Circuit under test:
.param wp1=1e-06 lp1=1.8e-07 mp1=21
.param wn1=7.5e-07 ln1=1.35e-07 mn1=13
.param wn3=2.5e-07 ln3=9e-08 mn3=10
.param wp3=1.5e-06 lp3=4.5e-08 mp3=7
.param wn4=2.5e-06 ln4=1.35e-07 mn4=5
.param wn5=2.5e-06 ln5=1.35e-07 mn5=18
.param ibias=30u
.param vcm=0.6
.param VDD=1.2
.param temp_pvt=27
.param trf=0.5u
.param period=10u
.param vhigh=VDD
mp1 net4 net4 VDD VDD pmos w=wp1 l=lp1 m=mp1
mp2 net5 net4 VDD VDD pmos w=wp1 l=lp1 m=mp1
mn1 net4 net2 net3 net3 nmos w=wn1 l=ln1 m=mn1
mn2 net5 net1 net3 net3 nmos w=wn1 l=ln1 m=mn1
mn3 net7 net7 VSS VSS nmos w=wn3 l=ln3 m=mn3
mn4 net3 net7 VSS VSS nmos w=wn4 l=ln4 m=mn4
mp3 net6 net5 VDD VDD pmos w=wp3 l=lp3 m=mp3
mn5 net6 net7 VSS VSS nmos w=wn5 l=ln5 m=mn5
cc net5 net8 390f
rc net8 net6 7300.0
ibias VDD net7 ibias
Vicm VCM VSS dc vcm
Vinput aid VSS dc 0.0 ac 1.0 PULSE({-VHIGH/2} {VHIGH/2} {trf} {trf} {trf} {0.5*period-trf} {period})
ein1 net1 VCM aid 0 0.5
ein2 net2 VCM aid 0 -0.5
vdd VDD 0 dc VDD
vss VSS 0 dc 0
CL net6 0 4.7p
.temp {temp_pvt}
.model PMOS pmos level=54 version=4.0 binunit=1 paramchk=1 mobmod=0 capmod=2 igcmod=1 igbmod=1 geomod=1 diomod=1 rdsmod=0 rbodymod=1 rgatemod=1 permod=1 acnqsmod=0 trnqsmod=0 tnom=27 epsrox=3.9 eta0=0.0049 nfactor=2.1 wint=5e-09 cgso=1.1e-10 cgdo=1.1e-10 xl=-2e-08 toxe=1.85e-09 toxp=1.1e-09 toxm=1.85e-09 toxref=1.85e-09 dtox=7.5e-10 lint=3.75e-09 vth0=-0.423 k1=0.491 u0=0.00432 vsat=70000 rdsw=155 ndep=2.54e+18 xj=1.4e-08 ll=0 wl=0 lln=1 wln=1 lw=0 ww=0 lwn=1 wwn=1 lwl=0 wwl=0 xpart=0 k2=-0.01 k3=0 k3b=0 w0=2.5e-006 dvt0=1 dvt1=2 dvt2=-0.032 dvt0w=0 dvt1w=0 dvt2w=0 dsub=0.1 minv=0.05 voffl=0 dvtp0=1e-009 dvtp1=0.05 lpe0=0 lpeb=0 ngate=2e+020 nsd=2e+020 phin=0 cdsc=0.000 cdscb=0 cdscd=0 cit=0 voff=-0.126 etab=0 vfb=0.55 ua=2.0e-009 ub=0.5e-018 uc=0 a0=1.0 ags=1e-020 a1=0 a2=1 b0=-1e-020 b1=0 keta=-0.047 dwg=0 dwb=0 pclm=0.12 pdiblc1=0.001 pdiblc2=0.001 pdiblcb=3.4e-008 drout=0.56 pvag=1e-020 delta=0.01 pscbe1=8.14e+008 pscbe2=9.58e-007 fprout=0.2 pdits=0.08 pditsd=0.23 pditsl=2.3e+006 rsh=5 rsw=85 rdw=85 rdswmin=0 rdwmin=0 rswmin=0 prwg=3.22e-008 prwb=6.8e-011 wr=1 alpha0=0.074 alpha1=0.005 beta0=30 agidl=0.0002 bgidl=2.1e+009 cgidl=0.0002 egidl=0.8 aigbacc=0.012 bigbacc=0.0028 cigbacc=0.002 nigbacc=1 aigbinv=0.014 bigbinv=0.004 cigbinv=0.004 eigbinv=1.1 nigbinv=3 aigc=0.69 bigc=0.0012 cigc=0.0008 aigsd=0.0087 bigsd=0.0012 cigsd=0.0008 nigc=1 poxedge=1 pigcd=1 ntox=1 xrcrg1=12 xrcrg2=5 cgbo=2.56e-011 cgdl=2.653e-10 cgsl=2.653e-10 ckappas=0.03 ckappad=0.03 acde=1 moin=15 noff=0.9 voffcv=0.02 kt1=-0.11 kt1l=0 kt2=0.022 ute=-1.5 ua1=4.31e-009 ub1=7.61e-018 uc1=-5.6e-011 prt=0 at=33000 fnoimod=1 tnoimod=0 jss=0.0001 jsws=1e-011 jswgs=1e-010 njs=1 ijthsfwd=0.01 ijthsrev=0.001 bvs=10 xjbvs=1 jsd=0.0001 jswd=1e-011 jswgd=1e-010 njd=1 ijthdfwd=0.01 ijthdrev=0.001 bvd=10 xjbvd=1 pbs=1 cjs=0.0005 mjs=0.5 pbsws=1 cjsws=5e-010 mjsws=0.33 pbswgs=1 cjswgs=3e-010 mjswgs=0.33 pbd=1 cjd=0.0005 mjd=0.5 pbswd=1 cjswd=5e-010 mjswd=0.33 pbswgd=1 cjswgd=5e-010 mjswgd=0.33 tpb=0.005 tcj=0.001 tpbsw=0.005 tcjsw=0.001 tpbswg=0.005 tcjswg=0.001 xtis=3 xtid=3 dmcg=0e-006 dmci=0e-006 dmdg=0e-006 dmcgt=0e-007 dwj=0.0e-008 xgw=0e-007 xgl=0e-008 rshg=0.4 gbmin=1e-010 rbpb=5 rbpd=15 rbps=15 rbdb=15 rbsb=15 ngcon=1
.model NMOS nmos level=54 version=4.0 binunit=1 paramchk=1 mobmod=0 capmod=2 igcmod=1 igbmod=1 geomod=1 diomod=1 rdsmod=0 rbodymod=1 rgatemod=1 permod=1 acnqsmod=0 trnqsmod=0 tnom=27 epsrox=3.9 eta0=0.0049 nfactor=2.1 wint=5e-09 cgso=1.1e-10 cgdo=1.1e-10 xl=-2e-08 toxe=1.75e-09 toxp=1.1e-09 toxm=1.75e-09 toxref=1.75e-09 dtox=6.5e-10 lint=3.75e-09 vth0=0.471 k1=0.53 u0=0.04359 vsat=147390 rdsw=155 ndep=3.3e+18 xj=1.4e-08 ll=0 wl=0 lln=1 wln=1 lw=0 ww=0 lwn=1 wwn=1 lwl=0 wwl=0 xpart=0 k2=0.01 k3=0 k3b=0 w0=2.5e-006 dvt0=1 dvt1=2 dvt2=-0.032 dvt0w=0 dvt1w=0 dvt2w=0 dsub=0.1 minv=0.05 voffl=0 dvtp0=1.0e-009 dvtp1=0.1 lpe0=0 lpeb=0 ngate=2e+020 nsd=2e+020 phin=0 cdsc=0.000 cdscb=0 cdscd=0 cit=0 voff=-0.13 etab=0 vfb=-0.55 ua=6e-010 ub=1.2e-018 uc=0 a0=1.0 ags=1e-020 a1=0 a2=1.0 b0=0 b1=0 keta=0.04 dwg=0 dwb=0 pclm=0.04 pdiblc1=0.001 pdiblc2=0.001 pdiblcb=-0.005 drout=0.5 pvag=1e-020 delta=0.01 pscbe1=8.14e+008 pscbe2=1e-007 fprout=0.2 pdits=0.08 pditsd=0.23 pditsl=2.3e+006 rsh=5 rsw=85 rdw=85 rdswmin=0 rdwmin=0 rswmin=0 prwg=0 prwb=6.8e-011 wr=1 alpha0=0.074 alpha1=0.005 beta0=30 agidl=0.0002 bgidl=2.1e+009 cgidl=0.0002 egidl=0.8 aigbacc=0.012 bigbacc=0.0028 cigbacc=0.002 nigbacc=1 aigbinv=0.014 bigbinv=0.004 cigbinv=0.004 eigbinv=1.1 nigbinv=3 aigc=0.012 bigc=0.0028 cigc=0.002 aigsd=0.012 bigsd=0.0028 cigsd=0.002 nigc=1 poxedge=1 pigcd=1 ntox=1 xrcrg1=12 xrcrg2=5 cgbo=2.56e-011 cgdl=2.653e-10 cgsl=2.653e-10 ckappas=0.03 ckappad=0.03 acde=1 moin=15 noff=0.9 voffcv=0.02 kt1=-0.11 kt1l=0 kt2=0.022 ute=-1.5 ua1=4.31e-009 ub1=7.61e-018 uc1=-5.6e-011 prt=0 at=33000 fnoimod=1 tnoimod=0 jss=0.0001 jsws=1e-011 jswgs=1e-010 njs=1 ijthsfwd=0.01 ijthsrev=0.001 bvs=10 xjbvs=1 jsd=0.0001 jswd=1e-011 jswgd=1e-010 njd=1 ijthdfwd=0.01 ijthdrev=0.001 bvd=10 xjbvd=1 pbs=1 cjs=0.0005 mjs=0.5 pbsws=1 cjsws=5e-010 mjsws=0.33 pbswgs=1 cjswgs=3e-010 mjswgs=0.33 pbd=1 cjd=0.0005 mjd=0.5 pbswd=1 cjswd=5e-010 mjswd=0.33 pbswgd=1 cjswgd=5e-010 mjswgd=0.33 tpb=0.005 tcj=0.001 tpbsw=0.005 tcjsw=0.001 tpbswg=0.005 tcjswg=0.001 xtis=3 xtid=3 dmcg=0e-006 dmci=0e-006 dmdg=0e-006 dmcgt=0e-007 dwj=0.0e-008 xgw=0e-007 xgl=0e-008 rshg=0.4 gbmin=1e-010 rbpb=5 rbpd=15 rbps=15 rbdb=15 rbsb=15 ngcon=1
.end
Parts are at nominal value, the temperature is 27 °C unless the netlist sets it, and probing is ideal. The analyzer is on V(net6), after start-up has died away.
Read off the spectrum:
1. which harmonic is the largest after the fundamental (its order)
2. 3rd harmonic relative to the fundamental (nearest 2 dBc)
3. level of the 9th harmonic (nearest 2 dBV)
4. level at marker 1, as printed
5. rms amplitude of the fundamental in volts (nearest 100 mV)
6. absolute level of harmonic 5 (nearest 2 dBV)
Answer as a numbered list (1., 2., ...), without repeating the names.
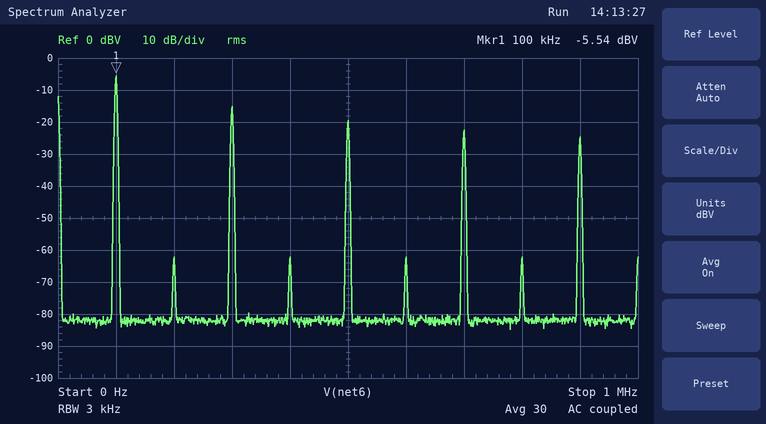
1. 3
2. -10 dBc
3. -24 dBV
4. -5.54 dBV
5. 500 mV
6. -20 dBV
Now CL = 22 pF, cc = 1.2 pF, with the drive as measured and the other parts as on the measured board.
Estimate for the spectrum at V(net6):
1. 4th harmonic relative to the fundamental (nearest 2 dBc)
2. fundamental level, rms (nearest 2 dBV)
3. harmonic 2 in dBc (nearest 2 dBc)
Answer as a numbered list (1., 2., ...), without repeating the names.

1. -40 dBc
2. -6 dBV
3. -40 dBc
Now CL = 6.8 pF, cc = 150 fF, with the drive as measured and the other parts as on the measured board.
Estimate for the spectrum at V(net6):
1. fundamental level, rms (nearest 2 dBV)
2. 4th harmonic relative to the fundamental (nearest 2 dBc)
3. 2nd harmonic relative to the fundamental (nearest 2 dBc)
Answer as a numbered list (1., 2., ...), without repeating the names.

1. -6 dBV
2. -52 dBc
3. -52 dBc
